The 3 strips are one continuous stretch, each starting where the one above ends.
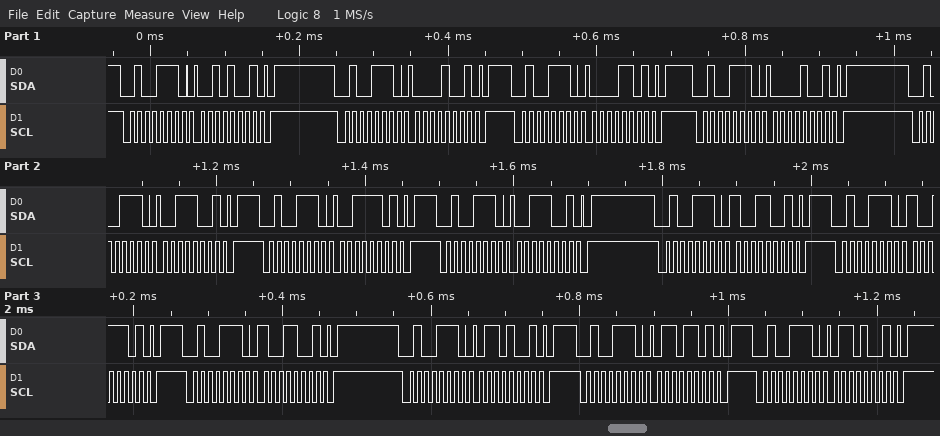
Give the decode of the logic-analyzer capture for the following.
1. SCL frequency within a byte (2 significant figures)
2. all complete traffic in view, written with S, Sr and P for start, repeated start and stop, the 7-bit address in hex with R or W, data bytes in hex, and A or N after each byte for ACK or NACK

100 kHz
S 27W A 29 A P S 27W A 09 A P S 27W A 0D A P S 27W A 09 A P S 27W A 39 A P S 27W A 3D A P S 27W A 39 A P S 27W A 99 A P S 27W A 9D A P S 27W A 99 A P S 27W A 69 A P S 27W A 6D A P S 27W A 69 A P
